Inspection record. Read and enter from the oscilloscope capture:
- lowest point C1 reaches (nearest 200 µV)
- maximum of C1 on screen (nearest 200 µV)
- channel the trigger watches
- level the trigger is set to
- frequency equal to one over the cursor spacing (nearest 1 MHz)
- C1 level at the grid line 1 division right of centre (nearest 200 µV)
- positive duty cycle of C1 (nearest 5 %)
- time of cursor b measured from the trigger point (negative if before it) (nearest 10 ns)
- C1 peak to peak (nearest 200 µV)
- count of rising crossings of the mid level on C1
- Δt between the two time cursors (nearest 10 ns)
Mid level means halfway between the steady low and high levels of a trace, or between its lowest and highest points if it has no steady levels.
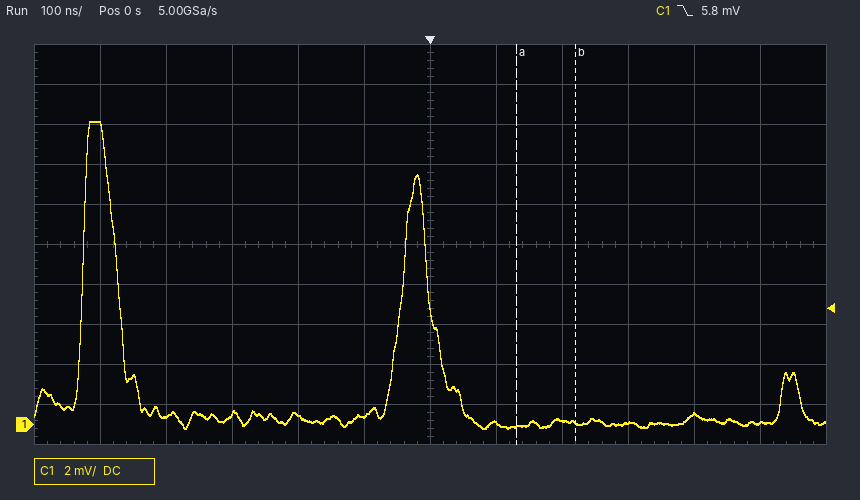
-200 µV
15.2 mV
C1
5.8 mV
11 MHz
0.0 mV
10 %
+220 ns
15.4 mV
2
90 ns
